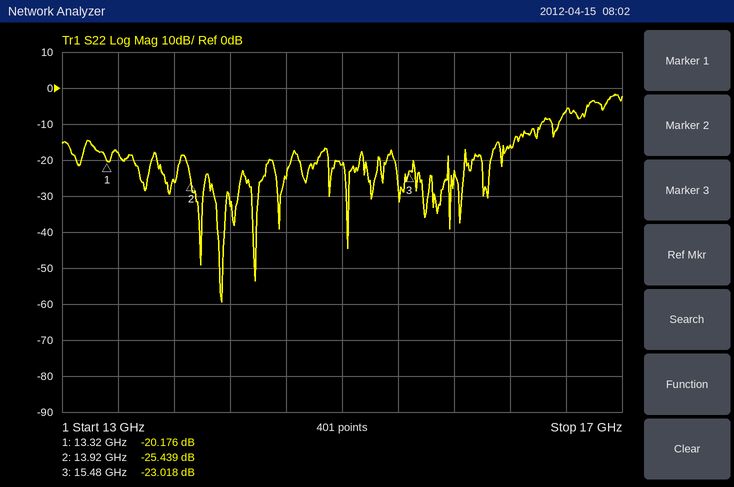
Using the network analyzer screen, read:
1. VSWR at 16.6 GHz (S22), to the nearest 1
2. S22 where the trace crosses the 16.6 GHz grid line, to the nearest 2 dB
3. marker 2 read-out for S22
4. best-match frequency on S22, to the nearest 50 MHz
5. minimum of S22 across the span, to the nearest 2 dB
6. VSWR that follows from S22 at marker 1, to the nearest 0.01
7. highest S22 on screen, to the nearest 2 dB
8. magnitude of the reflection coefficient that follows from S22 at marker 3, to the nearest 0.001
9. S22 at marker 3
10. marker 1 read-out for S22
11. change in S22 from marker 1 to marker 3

3
-6 dB
-25.439 dB
14.15 GHz
-60 dB
1.22
-2 dB
0.071
-23.018 dB
-20.176 dB
-2.842 dB
